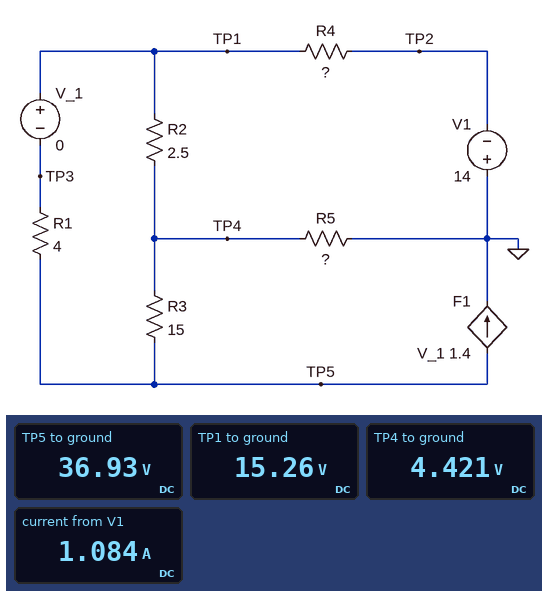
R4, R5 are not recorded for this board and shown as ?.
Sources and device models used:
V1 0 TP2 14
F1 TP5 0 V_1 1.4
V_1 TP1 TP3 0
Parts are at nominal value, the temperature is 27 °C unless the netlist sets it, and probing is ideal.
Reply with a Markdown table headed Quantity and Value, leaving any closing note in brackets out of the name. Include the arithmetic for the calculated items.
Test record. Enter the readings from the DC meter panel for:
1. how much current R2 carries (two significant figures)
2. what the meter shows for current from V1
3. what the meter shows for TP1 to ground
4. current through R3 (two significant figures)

| Quantity | Value |
|---|---|
| how much current R2 carries | (15.26 V - 4.421 V) / 2.5 Ω = 4.3 A |
| what the meter shows for current from V1 | 1.084 A |
| what the meter shows for TP1 to ground | 15.26 V |
| current through R3 | (36.93 V - 4.421 V) / 15 Ω = 2.2 A |
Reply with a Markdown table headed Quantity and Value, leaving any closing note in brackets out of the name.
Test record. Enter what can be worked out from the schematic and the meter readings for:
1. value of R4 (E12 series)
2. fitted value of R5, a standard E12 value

| Quantity | Value |
|---|---|
| value of R4 | 27 Ω |
| fitted value of R5, a standard E12 value | 0.68 Ω |
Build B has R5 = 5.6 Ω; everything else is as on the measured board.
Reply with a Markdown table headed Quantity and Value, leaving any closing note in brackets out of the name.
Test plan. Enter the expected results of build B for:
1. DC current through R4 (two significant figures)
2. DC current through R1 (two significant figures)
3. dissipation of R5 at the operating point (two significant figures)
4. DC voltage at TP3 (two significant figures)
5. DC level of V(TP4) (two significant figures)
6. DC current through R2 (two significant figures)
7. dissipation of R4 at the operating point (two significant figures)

| Quantity | Value |
|---|---|
| DC current through R4 | 840 mA |
| DC current through R1 | 4.2 A |
| dissipation of R5 at the operating point | 140 W |
| DC voltage at TP3 | -37 V |
| DC level of V(TP4) | -28 V |
| DC current through R2 | 3.4 A |
| dissipation of R4 at the operating point | 19 W |
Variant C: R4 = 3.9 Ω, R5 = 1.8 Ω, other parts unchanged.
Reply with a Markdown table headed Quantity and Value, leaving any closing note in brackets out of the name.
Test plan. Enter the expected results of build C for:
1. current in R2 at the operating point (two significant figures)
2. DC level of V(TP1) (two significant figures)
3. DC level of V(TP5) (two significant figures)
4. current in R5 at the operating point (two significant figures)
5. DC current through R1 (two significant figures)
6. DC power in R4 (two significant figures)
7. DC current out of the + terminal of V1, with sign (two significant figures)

| Quantity | Value |
|---|---|
| current in R2 at the operating point | 3.3 A |
| DC level of V(TP1) | -17 V |
| DC level of V(TP5) | -34 V |
| current in R5 at the operating point | 5.0 A |
| DC current through R1 | 4.1 A |
| DC power in R4 | 2.7 W |
| DC current out of the + terminal of V1, with sign | -830 mA |
